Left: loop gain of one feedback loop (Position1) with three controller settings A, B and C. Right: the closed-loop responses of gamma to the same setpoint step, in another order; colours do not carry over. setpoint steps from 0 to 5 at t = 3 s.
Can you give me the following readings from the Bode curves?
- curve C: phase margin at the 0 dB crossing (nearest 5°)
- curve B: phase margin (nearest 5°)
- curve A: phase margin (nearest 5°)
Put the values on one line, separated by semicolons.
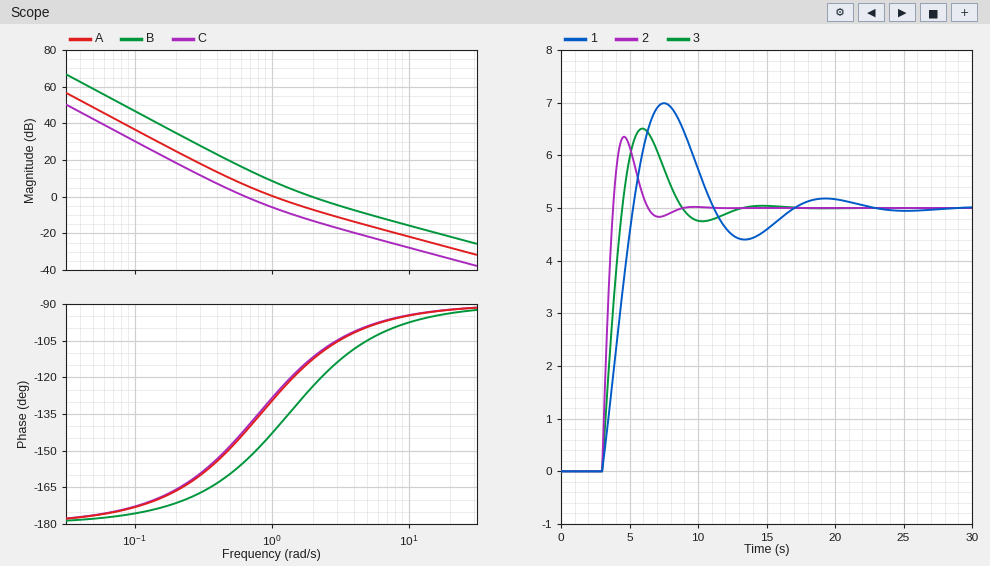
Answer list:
40°; 55°; 50°
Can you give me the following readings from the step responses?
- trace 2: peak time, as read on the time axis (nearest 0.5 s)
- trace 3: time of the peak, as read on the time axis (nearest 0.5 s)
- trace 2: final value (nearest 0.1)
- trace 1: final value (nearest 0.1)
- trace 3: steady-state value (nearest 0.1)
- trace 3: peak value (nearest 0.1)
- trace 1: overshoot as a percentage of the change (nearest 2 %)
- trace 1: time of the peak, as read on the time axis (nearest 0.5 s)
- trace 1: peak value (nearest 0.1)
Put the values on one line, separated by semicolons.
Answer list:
4.5 s; 6.0 s; 5.0; 5.0; 5.0; 6.5; 40 %; 7.5 s; 7.0
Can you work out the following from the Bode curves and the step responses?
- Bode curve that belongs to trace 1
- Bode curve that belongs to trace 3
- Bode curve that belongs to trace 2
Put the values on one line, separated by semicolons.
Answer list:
C; A; B
